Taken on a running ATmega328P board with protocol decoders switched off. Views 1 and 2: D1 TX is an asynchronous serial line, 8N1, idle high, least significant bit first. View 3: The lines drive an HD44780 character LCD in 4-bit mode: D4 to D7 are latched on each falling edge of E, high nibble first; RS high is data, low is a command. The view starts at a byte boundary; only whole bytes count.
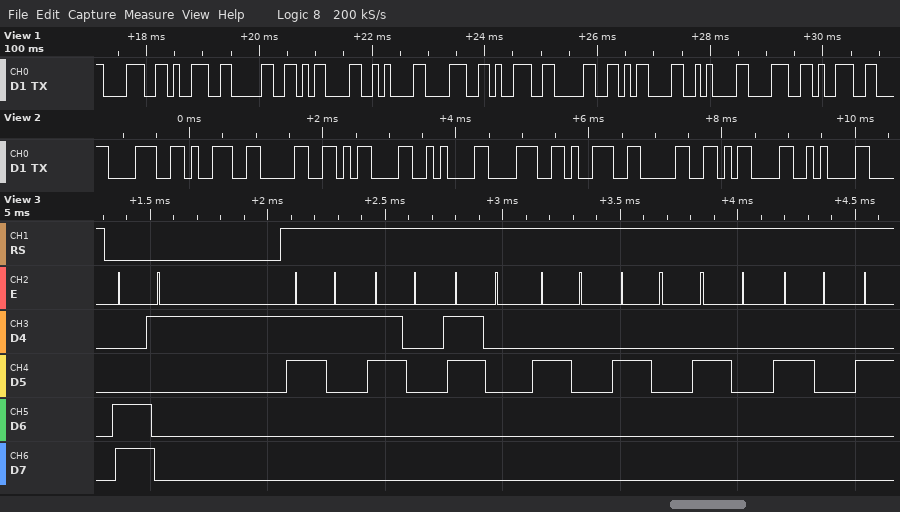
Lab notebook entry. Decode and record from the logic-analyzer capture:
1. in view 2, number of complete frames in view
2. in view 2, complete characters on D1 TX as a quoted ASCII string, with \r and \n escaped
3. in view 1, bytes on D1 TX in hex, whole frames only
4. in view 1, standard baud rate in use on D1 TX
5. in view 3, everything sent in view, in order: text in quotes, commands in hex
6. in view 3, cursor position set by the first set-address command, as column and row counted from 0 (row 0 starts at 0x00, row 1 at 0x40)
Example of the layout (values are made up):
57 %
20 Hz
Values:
10
"890\r\n890\r\n"
38 39 30 0D 0A 38 39 30 0D 0A 38 39
9600 baud
0xC1 "100    "
column 1, row 1
